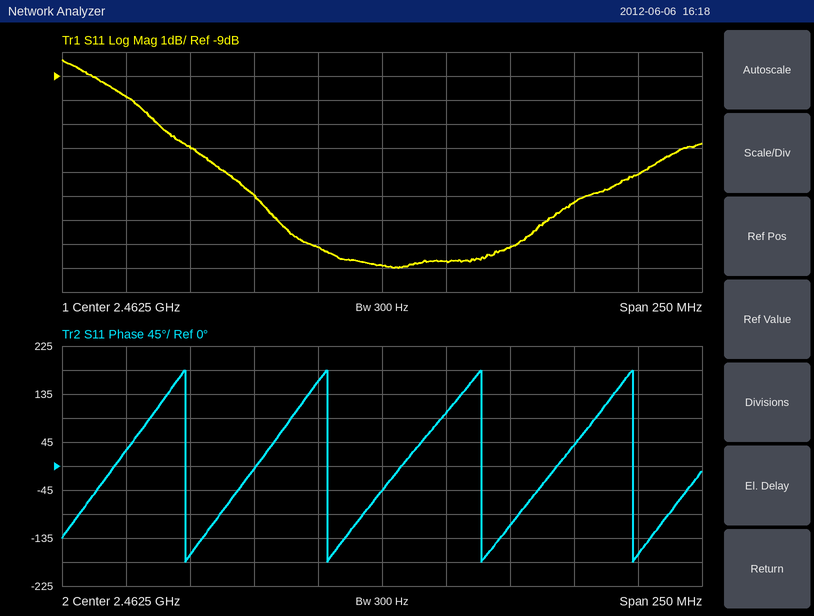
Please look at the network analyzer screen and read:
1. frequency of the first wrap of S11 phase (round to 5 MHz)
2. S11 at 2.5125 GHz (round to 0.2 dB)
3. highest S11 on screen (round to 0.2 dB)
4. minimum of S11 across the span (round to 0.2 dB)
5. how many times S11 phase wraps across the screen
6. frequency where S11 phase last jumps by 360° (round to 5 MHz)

2.385 GHz
-16.2 dB
-8.4 dB
-17.0 dB
4
2.560 GHz
